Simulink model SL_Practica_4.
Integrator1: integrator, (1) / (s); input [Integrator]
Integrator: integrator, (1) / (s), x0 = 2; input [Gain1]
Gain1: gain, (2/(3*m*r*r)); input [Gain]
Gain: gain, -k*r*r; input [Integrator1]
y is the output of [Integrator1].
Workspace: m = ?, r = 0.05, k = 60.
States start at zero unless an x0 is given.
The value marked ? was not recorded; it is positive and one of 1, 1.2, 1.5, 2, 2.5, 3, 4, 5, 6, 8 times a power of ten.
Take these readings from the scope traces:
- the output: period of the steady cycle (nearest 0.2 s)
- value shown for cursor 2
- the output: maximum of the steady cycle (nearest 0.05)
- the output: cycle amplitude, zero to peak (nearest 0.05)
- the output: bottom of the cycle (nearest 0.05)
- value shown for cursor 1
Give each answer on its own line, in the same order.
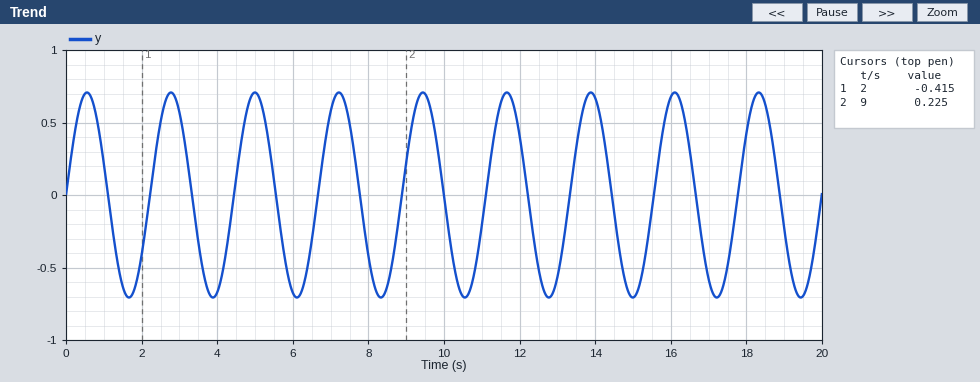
2.2 s
0.225
0.70
0.70
-0.70
-0.415
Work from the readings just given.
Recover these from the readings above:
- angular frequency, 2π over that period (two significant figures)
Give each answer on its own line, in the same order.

2.9 rad/s
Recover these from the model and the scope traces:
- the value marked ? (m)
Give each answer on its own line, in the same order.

5
